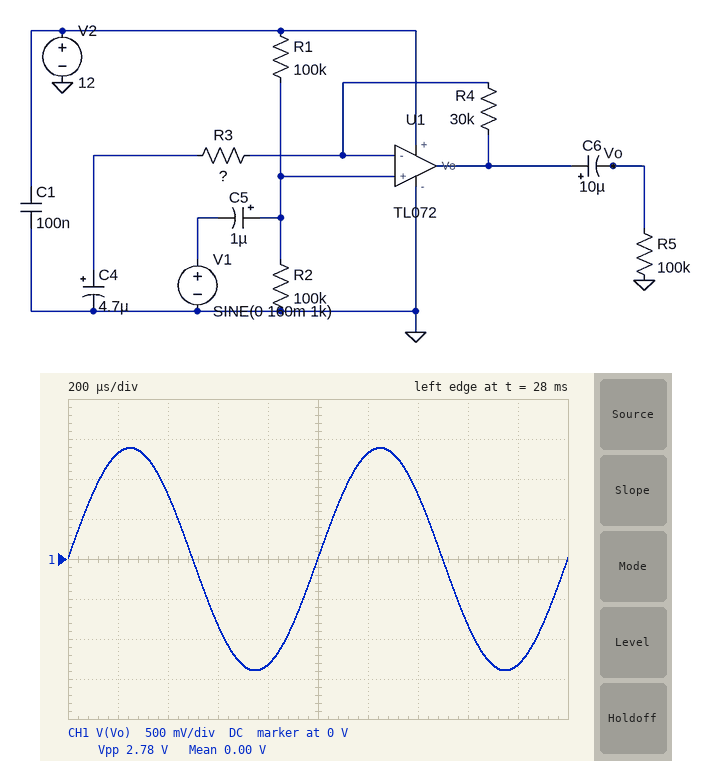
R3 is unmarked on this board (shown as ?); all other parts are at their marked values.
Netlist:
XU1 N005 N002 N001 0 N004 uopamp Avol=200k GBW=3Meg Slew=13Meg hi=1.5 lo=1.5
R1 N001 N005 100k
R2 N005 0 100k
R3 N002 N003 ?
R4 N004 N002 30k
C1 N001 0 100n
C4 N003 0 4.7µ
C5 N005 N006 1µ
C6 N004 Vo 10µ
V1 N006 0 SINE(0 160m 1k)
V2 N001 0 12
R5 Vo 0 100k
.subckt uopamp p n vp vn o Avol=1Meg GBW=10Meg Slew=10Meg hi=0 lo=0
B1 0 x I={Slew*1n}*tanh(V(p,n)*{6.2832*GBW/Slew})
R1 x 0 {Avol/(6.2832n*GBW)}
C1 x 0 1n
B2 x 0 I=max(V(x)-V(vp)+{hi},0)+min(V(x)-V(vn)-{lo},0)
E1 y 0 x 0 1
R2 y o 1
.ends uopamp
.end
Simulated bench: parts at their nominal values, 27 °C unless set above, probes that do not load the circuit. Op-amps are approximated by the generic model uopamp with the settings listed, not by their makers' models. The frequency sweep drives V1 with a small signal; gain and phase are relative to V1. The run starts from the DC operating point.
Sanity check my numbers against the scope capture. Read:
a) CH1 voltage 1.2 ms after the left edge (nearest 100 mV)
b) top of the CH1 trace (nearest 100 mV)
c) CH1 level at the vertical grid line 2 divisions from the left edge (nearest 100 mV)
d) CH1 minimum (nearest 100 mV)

1.3 V
1.4 V
800 mV
-1.4 V
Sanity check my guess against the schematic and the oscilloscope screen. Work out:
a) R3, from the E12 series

3.9 kΩ
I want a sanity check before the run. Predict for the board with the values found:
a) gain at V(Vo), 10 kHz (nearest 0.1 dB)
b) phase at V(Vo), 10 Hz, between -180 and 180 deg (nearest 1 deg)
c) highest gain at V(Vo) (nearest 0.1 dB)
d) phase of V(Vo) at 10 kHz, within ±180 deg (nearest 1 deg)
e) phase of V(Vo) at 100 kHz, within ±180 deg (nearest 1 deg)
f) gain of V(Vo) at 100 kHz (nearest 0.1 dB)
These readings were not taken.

18.8 dB
54 deg
18.8 dB
-2 deg
-16 deg
18.4 dB
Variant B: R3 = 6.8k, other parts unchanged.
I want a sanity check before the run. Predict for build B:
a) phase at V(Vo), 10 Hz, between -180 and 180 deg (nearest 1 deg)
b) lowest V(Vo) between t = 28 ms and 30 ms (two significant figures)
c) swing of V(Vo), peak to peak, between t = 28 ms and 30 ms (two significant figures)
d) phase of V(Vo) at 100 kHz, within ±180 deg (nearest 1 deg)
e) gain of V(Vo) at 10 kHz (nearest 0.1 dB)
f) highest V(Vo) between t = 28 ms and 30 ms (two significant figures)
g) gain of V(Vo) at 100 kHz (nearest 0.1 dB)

40 deg
-870 mV
1.7 V
-10 deg
14.7 dB
860 mV
14.5 dB
